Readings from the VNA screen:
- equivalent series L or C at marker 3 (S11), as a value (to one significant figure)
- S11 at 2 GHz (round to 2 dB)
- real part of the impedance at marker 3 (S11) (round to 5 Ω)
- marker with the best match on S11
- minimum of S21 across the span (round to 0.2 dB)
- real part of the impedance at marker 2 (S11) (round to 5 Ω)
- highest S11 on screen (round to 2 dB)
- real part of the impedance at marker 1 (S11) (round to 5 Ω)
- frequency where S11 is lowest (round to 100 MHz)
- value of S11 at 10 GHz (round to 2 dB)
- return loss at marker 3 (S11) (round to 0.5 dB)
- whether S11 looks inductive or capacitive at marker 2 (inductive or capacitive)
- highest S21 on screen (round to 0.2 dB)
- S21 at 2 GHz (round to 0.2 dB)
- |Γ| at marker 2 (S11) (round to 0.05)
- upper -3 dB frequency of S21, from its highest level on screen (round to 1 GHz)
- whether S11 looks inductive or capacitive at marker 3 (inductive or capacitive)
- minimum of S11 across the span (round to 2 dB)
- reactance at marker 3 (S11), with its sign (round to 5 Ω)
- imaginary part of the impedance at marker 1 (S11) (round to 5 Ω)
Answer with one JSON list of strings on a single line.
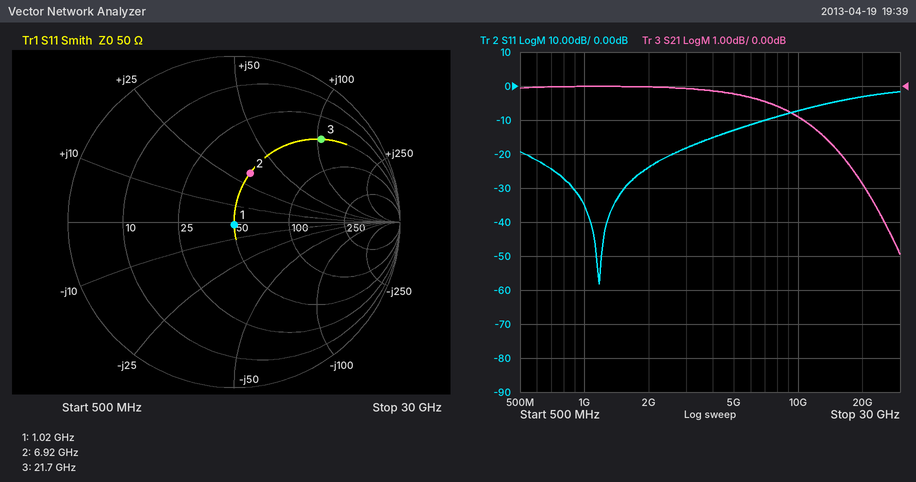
["800 pH", "-24 dB", "50 Ω", "marker 1", "-5.0 dB", "50 Ω", "-2 dB", "50 Ω", "1.2 GHz", "-8 dB", "3.0 dB", "inductive", "0.0 dB", "0.0 dB", "0.30", "21 GHz", "inductive", "-58 dB", "+105 Ω", "0 Ω"]
